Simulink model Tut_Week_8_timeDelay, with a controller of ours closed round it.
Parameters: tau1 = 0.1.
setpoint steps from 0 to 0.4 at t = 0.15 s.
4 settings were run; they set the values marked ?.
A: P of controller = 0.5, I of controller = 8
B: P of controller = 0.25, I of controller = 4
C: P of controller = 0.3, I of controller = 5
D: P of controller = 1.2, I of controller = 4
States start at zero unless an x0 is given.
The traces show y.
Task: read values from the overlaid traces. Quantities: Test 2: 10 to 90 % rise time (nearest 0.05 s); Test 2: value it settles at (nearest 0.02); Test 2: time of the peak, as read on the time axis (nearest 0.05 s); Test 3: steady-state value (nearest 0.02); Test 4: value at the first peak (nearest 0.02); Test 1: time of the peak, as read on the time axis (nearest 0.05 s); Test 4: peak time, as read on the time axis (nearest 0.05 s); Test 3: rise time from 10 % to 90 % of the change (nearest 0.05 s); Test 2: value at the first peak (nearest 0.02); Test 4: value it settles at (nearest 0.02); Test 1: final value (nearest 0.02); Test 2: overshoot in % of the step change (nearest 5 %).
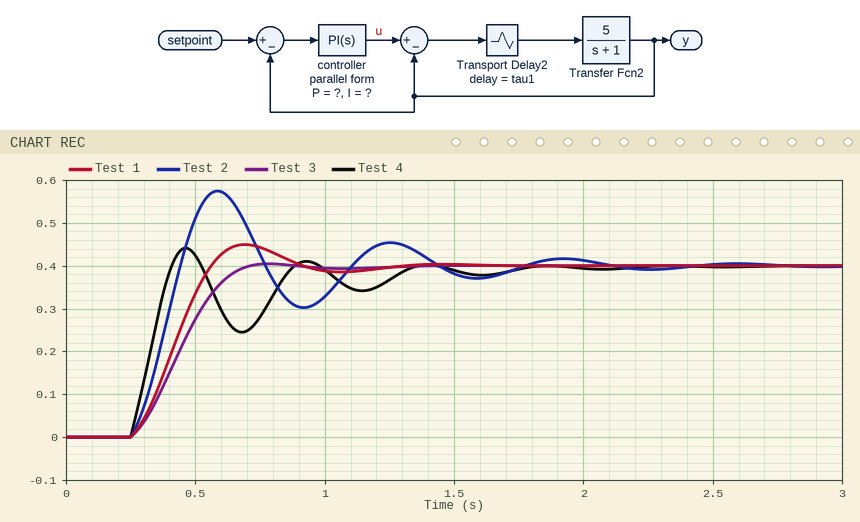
0.15 s
0.40
0.60 s
0.40
0.44
0.70 s
0.45 s
0.30 s
0.58
0.40
0.40
45 %
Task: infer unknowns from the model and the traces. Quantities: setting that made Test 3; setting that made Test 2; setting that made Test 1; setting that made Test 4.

B
A
C
D
